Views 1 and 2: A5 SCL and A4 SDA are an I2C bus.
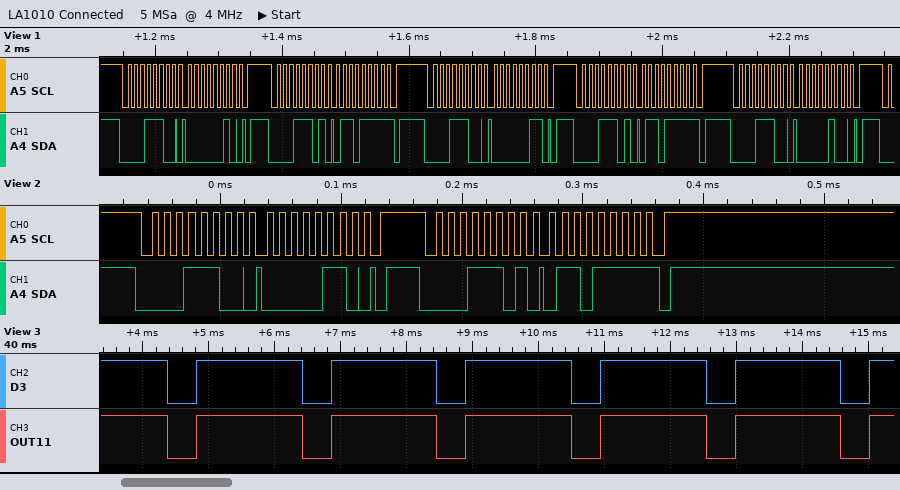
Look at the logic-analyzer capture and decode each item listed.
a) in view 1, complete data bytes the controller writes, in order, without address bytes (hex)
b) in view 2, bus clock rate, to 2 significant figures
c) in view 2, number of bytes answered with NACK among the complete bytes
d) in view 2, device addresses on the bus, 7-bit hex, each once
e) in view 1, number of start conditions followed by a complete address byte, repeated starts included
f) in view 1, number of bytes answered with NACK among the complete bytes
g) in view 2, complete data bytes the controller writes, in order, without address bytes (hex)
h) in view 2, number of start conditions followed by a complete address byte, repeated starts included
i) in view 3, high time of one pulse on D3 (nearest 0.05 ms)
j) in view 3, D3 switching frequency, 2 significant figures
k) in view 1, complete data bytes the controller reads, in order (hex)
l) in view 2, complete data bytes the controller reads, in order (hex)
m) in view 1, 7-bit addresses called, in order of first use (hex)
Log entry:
02 03 04
100 kHz
1
0x0E
5
2
06
2
1.60 ms
490 Hz
6F 6F
6F
0x0E
